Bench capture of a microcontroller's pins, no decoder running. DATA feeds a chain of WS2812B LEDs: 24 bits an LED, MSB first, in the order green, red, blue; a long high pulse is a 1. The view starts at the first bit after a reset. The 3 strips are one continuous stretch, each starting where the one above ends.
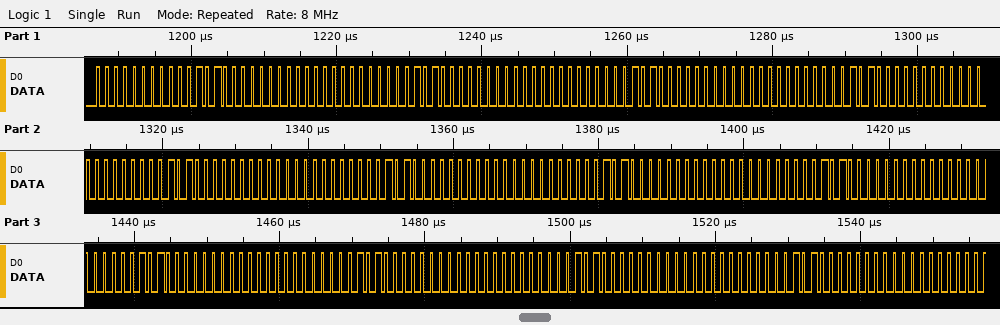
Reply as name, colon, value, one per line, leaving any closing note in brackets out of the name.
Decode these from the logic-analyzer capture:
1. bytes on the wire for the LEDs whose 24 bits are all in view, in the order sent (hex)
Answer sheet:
bytes on the wire for the LEDs whose 24 bits are all in view, in the order sent: 00 14 00 00 14 00 00 14 00 00 14 00 00 14 00 00 14 00 00 14 00 00 14 00 00 14 00 00 14 00 00 14 00 00 14 00
